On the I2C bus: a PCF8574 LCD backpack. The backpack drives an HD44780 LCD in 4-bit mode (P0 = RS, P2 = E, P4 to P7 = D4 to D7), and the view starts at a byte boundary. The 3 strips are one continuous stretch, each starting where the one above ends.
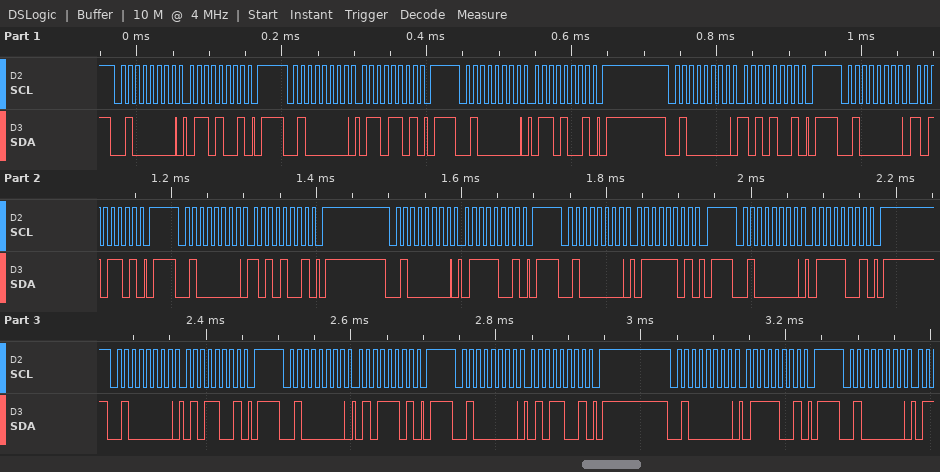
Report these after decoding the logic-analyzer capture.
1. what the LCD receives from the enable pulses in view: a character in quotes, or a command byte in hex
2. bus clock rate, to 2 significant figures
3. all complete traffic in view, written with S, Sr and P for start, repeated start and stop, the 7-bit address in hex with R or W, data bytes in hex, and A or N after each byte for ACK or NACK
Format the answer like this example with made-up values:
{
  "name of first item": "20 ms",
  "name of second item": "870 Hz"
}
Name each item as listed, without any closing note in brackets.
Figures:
{
  "what the LCD receives from the enable pulses in view: a character in quotes, or a command byte in hex": "'j' 'u'",
  "bus clock rate, to 2 significant figures": "100 kHz",
  "all complete traffic in view, written with S, Sr and P for start, repeated start and stop, the 7-bit address in hex with R or W, data bytes in hex, and A or N after each byte for ACK or NACK": "S 20W A 69 A P S 20W A 6D A P S 20W A 69 A P S 20W A A9 A P S 20W A AD A P S 20W A A9 A P S 20W A 79 A P S 20W A 7D A P S 20W A 79 A P S 20W A 59 A P S 20W A 5D A P S 20W A 59 A P S 20W A 79 A P S 20W A"
}
